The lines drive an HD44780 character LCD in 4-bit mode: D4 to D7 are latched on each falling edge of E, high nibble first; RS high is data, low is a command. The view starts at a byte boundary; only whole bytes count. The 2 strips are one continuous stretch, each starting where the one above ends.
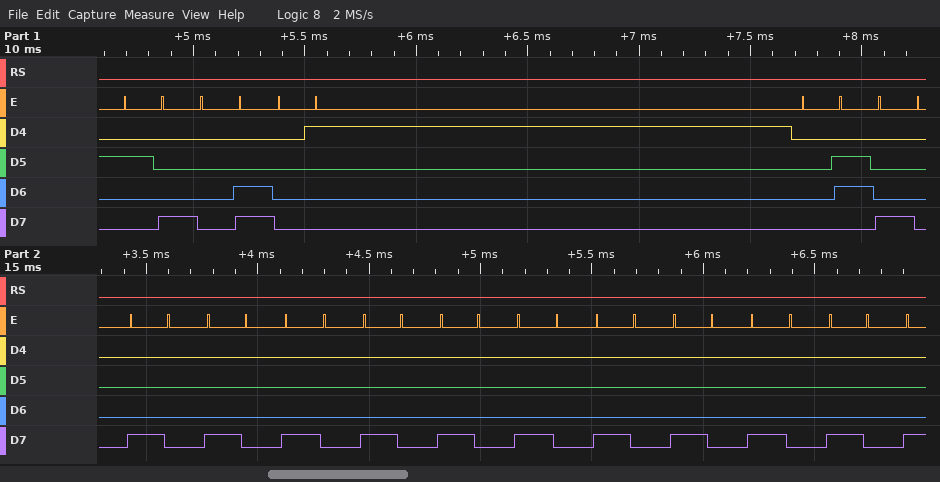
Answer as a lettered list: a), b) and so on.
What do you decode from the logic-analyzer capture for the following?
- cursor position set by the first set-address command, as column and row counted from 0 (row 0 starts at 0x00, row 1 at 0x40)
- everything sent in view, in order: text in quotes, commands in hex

a) column 0, row 0
b) 0x28 0x0C 0x01 0x06 0x80 0x80 0x80 0x80 0x80 0x80 0x80 0x80 0x80 0x80 0x80
